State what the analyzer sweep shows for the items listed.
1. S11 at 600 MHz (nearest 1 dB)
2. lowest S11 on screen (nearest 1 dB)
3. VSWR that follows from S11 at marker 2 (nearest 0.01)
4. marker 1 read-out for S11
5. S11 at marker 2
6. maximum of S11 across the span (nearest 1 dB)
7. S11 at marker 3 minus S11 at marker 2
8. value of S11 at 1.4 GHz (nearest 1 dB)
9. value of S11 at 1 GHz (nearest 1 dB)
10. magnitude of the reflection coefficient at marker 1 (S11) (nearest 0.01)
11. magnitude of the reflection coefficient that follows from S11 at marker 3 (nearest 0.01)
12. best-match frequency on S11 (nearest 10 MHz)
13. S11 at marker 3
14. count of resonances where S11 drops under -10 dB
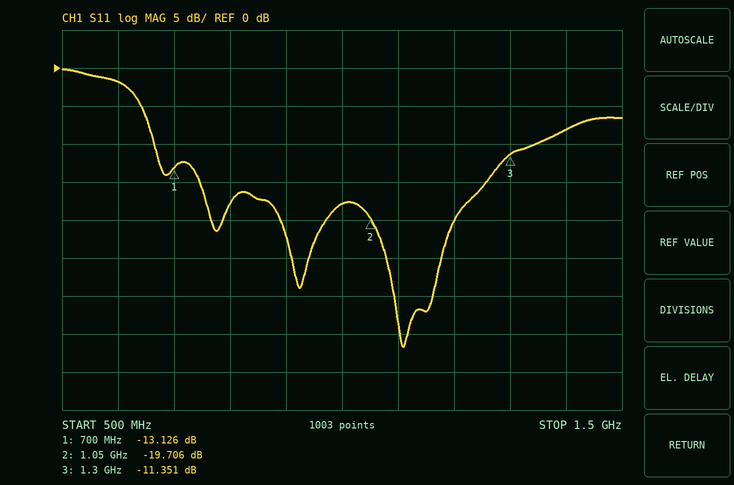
-2 dB
-37 dB
1.23
-13.126 dB
-19.706 dB
0 dB
8.355 dB
-8 dB
-18 dB
0.22
0.27
1.11 GHz
-11.351 dB
3
